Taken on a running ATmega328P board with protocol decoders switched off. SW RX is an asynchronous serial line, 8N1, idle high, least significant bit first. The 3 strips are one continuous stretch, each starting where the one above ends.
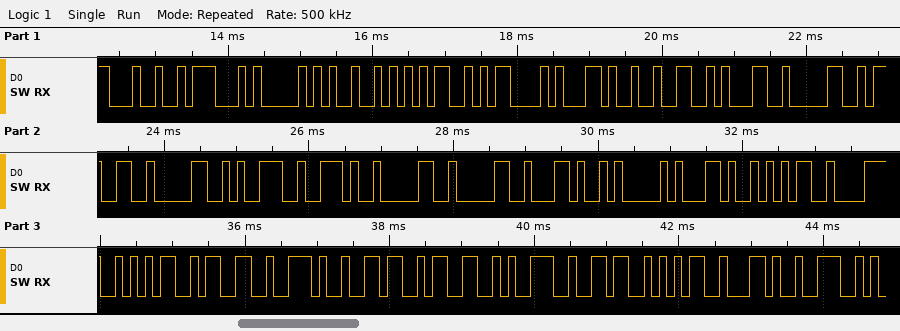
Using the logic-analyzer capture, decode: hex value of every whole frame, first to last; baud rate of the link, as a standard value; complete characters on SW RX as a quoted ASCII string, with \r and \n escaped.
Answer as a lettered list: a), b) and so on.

a) 24 47 50 52 4D 43 2C 32 31 30 33 30 39 2E 30 30 2C 41 2C 35 38 35 33 2E 36 33 39 36 35 2C 4E
b) 9600 baud
c) "$GPRMC,210309.00,A,5853.63965,N"
